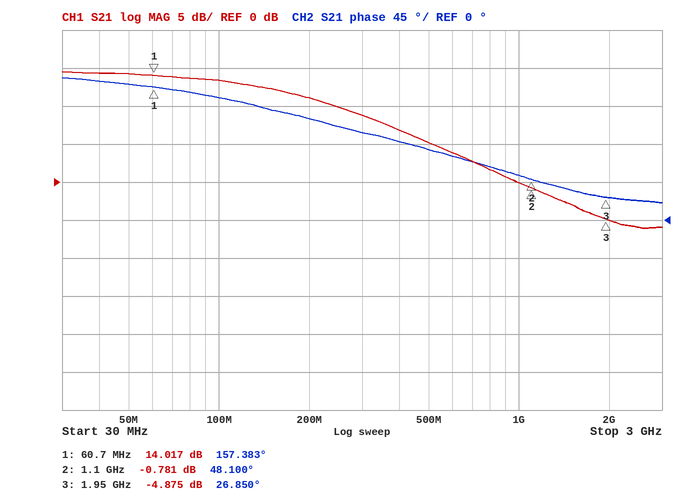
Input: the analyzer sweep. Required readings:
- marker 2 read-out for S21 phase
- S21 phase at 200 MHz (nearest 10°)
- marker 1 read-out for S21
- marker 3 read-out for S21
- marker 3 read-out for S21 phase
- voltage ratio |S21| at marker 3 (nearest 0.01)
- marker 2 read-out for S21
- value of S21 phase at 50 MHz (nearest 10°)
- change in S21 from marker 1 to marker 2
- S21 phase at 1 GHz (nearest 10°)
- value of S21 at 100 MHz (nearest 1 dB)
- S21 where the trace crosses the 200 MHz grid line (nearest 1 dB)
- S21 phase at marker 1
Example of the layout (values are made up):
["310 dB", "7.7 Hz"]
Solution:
["48.100°", "120°", "14.017 dB", "-4.875 dB", "26.850°", "0.57", "-0.781 dB", "160°", "-14.798 dB", "50°", "13 dB", "11 dB", "157.383°"]
